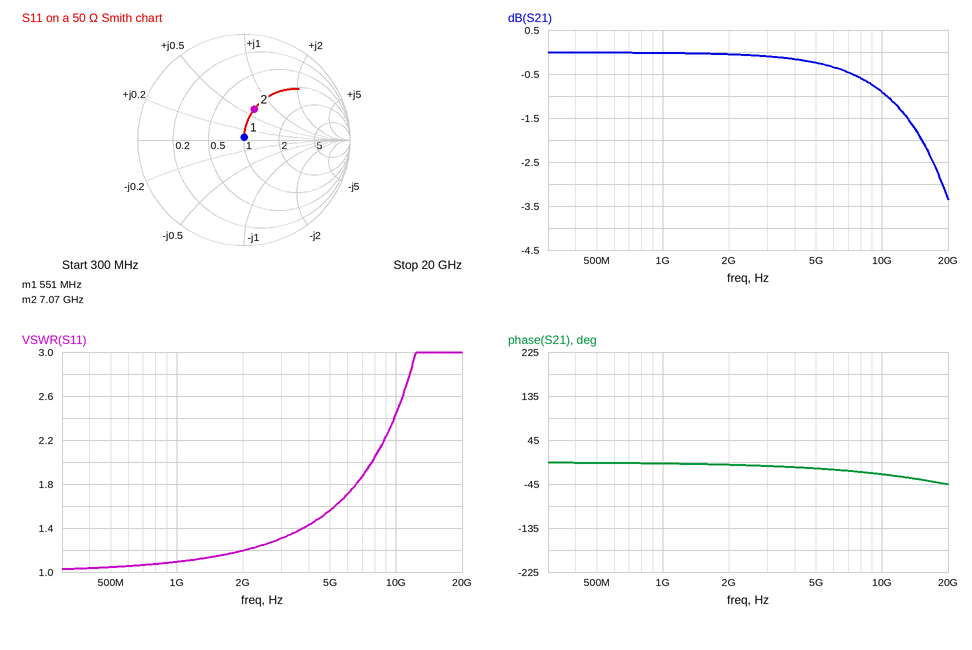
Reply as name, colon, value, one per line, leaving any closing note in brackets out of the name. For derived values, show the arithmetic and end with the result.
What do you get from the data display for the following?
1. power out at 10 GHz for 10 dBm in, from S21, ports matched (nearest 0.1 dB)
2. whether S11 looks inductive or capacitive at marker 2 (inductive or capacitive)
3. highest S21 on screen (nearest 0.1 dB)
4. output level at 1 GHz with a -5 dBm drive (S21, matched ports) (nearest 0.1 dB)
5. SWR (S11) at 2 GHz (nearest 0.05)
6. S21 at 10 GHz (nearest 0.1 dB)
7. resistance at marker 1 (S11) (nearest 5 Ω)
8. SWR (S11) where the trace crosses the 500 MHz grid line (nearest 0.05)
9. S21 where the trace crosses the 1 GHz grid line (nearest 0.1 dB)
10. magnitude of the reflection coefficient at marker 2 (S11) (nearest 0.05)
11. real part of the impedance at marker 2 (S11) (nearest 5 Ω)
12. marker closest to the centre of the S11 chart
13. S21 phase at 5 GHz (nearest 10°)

power out at 10 GHz for 10 dBm in, from S21, ports matched: 10 dBm + (-0.9 dB) = 9.1 dBm
whether S11 looks inductive or capacitive at marker 2: inductive
highest S21 on screen: 0.0 dB
output level at 1 GHz with a -5 dBm drive (S21, matched ports): -5 dBm + (0.0 dB) = -5.0 dBm
SWR (S11) at 2 GHz: 1.20
S21 at 10 GHz: -0.9 dB
resistance at marker 1 (S11): 50 Ω
SWR (S11) where the trace crosses the 500 MHz grid line: 1.05
S21 where the trace crosses the 1 GHz grid line: 0.0 dB
magnitude of the reflection coefficient at marker 2 (S11): 0.30
real part of the impedance at marker 2 (S11): 50 Ω
marker closest to the centre of the S11 chart: marker 1
S21 phase at 5 GHz: -10°
